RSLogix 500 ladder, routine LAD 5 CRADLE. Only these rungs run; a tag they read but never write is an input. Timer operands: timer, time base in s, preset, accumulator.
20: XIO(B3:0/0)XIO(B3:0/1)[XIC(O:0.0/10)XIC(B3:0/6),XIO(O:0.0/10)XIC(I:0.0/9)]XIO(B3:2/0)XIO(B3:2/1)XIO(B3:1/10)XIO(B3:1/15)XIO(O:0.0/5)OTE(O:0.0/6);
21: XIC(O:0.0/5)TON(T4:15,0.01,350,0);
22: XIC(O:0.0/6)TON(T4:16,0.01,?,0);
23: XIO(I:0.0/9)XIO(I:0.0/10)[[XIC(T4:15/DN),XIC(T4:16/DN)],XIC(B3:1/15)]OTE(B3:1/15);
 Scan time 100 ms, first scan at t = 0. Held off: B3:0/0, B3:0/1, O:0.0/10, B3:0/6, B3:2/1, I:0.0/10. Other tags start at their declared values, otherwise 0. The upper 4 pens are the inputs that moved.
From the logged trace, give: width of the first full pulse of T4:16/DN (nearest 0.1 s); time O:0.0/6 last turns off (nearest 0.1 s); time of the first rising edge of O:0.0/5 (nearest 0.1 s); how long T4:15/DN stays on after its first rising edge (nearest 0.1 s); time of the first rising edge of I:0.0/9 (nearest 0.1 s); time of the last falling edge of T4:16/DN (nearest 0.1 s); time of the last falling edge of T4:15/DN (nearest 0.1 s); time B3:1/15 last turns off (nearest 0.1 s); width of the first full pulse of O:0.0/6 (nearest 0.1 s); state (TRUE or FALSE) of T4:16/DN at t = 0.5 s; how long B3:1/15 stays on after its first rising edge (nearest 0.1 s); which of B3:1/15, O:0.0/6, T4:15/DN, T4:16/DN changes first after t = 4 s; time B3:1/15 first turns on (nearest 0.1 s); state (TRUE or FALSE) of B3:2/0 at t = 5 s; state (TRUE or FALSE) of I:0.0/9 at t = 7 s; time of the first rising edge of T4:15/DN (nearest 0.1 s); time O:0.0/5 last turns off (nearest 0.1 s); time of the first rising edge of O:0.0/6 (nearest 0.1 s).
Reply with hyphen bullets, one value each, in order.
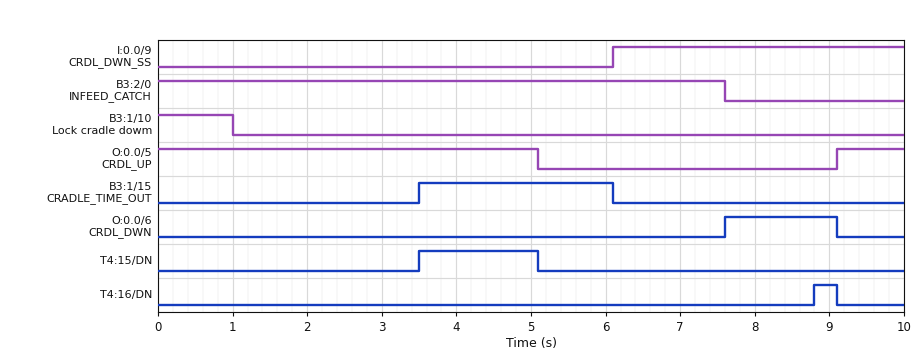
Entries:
- 0.3 s
- 9.1 s
- 9.1 s
- 1.6 s
- 6.1 s
- 9.1 s
- 5.1 s
- 6.1 s
- 1.5 s
- FALSE
- 2.6 s
- T4:15/DN
- 3.5 s
- TRUE
- TRUE
- 3.5 s
- 5.1 s
- 7.6 s
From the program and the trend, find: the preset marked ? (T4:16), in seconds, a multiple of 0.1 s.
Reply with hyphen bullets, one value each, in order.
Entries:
- 1.2 s
